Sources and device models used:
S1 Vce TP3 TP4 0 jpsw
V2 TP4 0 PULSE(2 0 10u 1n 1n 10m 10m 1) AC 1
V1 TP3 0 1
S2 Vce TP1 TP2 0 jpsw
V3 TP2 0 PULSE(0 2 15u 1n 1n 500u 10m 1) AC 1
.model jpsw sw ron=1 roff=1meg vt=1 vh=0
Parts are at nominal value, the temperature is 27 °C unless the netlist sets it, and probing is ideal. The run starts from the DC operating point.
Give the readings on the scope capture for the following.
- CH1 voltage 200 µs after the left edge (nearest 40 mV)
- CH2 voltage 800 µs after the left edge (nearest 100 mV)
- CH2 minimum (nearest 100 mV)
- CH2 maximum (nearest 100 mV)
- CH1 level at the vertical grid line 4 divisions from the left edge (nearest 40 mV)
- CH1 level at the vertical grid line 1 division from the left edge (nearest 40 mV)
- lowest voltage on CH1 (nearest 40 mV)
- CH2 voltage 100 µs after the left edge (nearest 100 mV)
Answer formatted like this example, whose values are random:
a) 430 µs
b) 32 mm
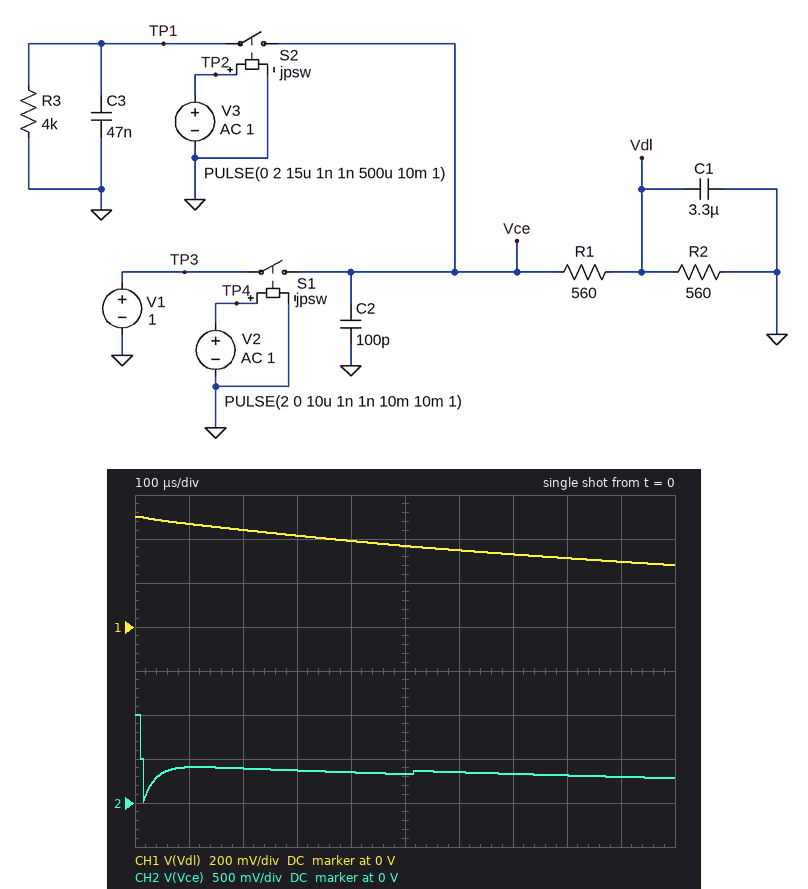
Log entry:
a) 440 mV
b) 300 mV
c) 0 V
d) 1.0 V
e) 400 mV
f) 480 mV
g) 280 mV
h) 400 mV
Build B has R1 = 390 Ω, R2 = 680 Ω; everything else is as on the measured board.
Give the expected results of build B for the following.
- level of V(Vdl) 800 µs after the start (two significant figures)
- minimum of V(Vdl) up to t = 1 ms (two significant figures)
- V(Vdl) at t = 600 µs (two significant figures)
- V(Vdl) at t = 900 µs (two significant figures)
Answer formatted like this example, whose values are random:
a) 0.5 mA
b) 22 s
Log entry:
a) 430 mV
b) 390 mV
c) 470 mV
d) 410 mV
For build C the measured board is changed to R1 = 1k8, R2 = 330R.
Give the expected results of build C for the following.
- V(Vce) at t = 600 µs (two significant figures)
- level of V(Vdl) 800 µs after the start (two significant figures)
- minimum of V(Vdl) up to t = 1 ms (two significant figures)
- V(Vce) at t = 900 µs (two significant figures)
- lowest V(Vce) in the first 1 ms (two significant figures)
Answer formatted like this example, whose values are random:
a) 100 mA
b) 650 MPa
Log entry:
a) 89 mV
b) 73 mV
c) 61 mV
d) 68 mV
e) 4.3 mV
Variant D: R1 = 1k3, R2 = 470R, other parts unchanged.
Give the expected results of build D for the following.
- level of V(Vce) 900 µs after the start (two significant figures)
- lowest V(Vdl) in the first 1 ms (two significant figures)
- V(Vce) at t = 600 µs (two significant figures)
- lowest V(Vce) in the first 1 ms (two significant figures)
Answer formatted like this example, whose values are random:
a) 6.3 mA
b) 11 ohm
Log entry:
a) 150 mV
b) 140 mV
c) 180 mV
d) 4.7 mV
